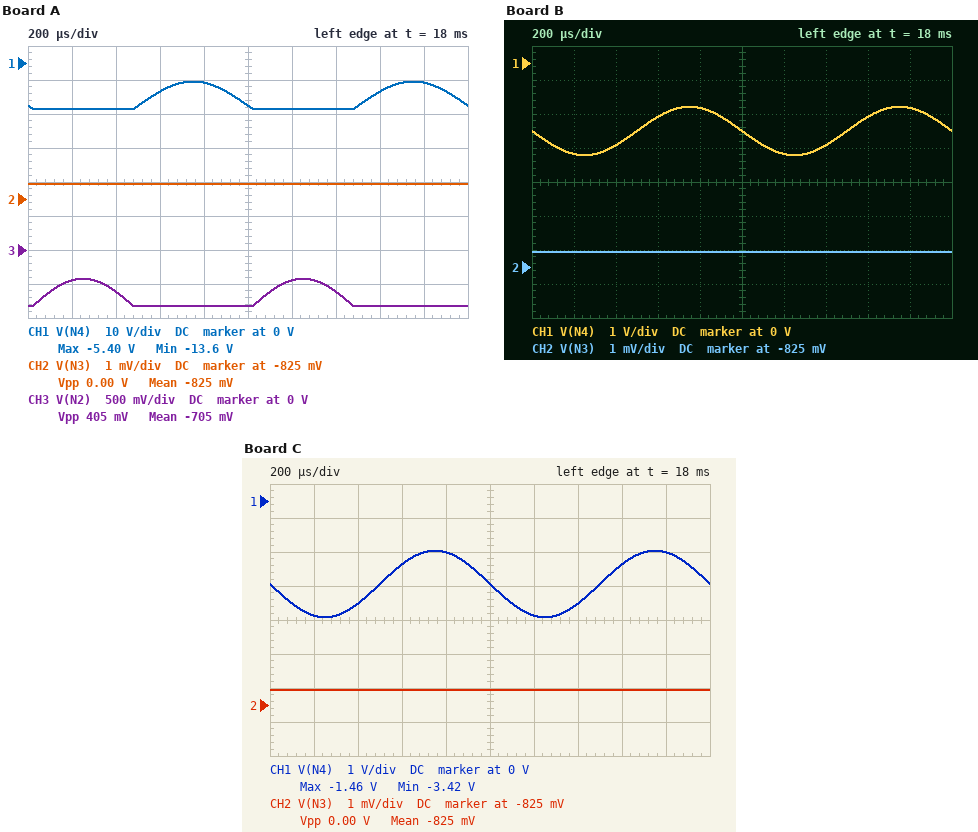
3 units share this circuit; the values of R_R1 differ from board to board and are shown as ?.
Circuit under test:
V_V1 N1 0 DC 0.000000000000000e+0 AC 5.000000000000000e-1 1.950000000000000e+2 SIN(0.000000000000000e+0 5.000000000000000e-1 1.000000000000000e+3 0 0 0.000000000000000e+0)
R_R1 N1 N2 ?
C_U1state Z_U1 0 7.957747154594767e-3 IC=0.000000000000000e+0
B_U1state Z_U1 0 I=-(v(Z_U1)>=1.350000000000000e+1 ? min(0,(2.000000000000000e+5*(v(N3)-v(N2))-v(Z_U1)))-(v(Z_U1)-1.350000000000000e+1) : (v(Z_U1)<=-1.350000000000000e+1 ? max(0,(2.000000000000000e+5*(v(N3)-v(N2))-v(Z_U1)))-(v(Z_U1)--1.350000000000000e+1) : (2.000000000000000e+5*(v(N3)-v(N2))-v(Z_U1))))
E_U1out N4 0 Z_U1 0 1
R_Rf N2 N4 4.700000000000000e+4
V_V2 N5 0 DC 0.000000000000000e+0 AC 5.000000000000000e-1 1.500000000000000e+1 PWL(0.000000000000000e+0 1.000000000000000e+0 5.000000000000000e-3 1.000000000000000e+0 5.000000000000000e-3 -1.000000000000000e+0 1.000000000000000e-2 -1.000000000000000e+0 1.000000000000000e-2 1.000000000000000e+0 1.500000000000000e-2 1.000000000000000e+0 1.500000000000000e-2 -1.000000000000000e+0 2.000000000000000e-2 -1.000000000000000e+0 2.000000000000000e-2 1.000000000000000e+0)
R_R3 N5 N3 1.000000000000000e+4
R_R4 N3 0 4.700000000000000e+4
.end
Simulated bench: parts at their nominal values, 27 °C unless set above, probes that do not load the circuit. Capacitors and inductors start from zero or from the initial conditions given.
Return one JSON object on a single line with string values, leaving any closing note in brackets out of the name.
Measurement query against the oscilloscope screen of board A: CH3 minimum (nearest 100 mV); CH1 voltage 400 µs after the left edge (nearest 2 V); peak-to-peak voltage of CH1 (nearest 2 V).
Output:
{"CH3 minimum": "-800 mV", "CH1 voltage 400 µs after the left edge": "-14 V", "peak-to-peak voltage of CH1": "8 V"}
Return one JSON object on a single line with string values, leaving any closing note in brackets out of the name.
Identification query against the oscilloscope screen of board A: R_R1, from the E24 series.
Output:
{"R_R1, from the E24 series": "3.3 kΩ"}
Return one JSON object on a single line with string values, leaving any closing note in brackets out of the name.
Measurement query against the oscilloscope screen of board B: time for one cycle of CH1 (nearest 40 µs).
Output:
{"time for one cycle of CH1": "1.00 ms"}
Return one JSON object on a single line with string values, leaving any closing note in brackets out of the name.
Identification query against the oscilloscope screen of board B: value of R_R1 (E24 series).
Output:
{"value of R_R1": "33 kΩ"}
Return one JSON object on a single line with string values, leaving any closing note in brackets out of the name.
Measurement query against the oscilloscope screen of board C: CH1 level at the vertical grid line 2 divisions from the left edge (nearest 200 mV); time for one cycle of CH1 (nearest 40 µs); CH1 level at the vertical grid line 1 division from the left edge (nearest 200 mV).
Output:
{"CH1 level at the vertical grid line 2 divisions from the left edge": "-3.0 V", "time for one cycle of CH1": "1.00 ms", "CH1 level at the vertical grid line 1 division from the left edge": "-3.4 V"}
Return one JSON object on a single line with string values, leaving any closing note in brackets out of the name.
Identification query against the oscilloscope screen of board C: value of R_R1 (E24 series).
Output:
{"value of R_R1": "24 kΩ"}
